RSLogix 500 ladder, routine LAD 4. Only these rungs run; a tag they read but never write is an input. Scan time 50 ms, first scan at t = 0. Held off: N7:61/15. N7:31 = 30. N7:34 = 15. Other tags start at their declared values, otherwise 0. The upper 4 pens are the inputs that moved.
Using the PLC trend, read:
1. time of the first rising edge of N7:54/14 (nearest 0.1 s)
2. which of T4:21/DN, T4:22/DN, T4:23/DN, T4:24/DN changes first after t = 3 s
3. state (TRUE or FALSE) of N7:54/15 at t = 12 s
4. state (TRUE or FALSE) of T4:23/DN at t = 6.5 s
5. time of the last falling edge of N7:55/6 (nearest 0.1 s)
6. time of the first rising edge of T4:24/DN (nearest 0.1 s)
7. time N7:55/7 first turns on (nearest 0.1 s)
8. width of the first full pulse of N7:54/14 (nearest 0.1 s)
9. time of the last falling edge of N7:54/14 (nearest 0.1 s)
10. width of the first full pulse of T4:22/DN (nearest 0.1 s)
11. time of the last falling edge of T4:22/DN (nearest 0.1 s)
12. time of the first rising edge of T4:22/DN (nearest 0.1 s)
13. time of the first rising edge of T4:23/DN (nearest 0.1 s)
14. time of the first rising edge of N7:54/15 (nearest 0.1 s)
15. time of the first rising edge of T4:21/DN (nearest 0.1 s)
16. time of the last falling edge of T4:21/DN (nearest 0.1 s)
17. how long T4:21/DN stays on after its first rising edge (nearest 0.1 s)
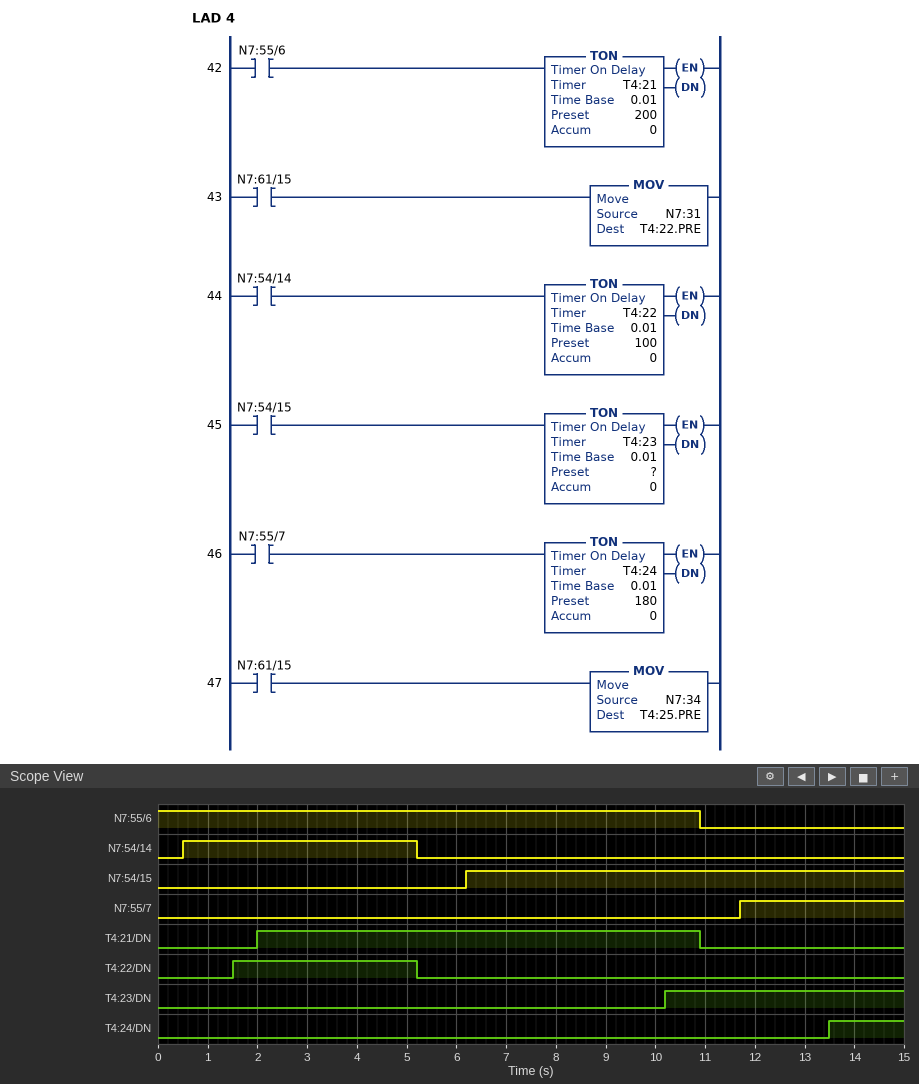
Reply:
0.5 s
T4:22/DN
TRUE
FALSE
10.9 s
13.5 s
11.7 s
4.7 s
5.2 s
3.7 s
5.2 s
1.5 s
10.2 s
6.2 s
2.0 s
10.9 s
8.9 s
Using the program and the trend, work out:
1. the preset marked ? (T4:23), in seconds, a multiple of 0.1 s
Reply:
4.0 s
